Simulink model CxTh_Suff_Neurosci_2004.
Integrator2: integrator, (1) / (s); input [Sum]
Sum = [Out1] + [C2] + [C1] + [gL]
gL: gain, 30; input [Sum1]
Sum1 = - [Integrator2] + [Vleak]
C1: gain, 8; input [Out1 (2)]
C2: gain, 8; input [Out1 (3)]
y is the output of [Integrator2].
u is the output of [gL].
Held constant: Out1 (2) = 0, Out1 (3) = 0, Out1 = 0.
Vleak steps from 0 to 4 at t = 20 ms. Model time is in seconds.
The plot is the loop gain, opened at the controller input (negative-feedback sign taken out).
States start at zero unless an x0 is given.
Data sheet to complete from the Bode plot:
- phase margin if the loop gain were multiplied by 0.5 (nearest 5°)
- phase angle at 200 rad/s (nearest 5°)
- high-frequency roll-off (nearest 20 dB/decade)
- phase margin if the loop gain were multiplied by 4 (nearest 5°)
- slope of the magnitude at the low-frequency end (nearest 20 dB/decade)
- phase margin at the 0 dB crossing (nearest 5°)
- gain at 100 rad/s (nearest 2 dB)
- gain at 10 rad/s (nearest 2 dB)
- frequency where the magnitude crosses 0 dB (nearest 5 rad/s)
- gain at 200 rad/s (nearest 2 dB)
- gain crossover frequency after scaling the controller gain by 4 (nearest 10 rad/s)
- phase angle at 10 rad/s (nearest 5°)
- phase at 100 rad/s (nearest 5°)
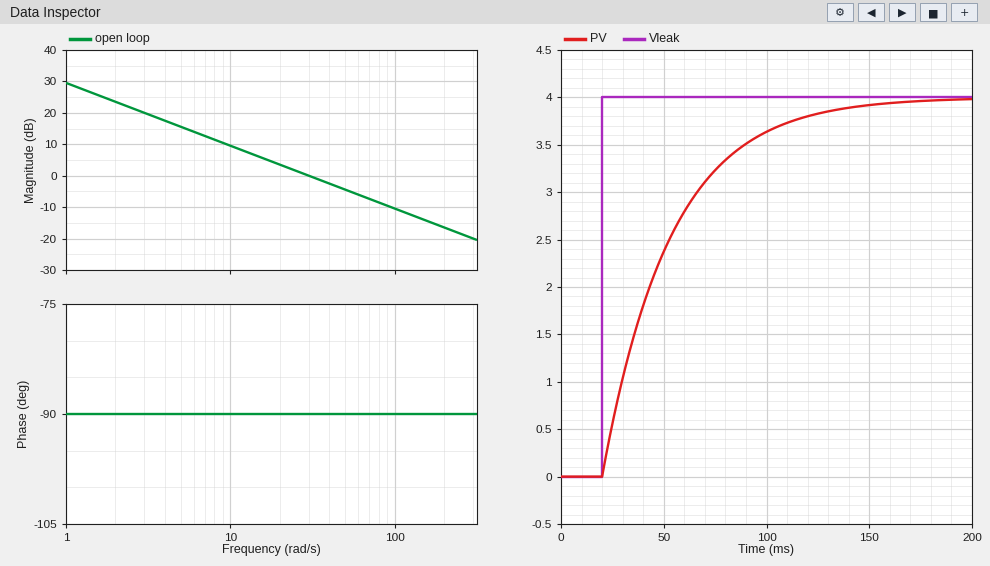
90°
-90°
-20 dB/decade
90°
-20 dB/decade
90°
-10 dB
10 dB
30 rad/s
-16 dB
120 rad/s
-90°
-90°
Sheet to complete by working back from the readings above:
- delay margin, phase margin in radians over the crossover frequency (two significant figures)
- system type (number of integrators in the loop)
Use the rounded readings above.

0.052 s
1
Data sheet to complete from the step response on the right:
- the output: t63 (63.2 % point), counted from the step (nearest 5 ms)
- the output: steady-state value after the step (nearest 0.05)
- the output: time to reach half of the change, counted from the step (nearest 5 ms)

35 ms
4.00
25 ms
